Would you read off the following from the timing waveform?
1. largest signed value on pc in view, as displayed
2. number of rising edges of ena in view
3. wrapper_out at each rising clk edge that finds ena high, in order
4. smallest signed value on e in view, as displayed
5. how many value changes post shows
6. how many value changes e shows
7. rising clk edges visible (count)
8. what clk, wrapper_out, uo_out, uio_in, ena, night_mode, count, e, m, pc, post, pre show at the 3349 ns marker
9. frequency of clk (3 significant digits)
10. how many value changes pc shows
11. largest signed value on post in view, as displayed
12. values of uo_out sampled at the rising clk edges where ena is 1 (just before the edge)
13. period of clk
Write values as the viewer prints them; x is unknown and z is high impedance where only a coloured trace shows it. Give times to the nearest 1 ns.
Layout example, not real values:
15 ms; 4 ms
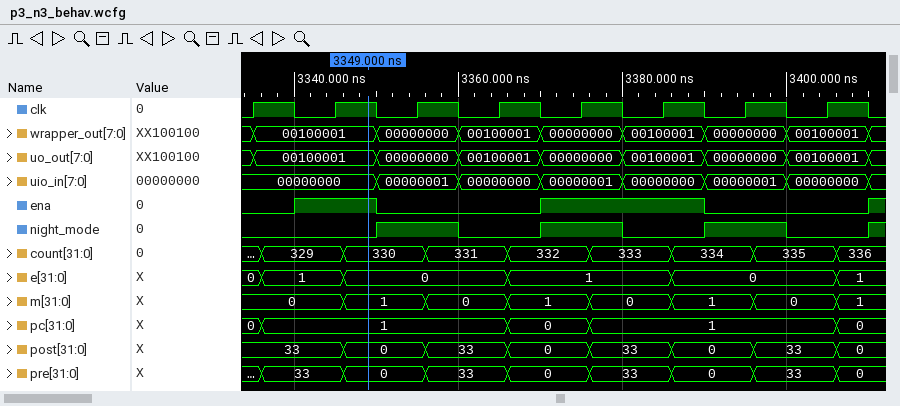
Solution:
1; 3; 00100001, 00000000, 00100001; 0; 7; 5; 8; clk=1, wrapper_out=00100001, uo_out=00100001, uio_in=00000000, ena=1, night_mode=0, count=330, e=0, m=1, pc=1, post=0, pre=0; 100 MHz; 4; 33; 00100001, 00000000, 00100001; 10 ns
